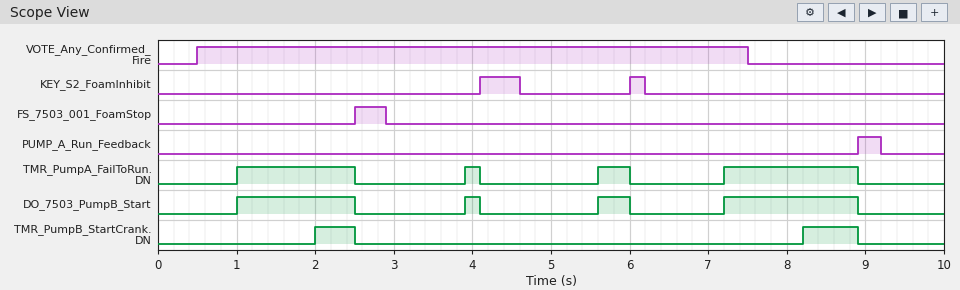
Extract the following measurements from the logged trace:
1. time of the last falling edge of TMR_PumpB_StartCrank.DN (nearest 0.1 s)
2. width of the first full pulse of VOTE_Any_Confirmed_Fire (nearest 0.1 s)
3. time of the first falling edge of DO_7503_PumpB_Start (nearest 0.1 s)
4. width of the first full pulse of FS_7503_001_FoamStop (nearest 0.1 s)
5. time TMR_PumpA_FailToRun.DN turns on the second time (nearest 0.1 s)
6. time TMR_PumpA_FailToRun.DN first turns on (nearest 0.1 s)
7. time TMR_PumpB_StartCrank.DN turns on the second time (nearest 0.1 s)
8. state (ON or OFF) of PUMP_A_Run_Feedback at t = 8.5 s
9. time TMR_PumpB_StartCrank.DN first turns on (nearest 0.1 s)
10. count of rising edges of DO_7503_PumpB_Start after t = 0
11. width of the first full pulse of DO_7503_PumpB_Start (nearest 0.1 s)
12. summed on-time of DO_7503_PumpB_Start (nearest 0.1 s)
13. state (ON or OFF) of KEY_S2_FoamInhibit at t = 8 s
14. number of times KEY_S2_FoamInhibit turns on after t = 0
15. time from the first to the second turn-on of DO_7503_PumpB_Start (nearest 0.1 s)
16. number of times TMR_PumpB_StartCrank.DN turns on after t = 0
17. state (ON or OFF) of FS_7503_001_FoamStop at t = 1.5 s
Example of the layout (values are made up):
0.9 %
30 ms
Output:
8.9 s
7.0 s
2.5 s
0.4 s
3.9 s
1.0 s
8.2 s
OFF
2.0 s
4
1.5 s
3.8 s
OFF
2
2.9 s
2
OFF
